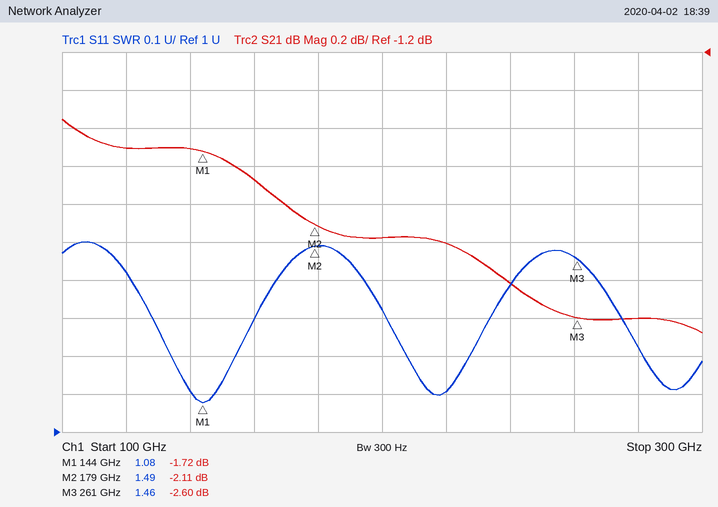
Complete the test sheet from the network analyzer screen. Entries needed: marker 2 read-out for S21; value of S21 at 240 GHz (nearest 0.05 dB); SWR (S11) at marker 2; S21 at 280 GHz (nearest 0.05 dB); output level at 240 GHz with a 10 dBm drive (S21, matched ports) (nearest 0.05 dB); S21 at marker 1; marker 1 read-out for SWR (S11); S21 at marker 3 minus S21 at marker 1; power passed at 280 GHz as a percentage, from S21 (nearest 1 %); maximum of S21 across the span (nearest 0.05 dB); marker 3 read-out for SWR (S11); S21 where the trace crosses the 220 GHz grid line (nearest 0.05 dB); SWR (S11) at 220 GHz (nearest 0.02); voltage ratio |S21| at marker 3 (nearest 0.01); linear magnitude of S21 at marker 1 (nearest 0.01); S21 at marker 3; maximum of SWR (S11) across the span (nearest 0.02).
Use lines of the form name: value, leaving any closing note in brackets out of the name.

marker 2 read-out for S21: -2.11 dB
value of S21 at 240 GHz: -2.40 dB
SWR (S11) at marker 2: 1.49
S21 at 280 GHz: -2.60 dB
output level at 240 GHz with a 10 dBm drive (S21, matched ports): 7.60 dBm
S21 at marker 1: -1.72 dB
marker 1 read-out for SWR: 1.08
S21 at marker 3 minus S21 at marker 1: -0.88 dB
power passed at 280 GHz as a percentage, from S21: 55 %
maximum of S21 across the span: -1.55 dB
marker 3 read-out for SWR: 1.46
S21 where the trace crosses the 220 GHz grid line: -2.20 dB
SWR (S11) at 220 GHz: 1.10
voltage ratio |S21| at marker 3: 0.74
linear magnitude of S21 at marker 1: 0.82
S21 at marker 3: -2.60 dB
maximum of SWR (S11) across the span: 1.50
